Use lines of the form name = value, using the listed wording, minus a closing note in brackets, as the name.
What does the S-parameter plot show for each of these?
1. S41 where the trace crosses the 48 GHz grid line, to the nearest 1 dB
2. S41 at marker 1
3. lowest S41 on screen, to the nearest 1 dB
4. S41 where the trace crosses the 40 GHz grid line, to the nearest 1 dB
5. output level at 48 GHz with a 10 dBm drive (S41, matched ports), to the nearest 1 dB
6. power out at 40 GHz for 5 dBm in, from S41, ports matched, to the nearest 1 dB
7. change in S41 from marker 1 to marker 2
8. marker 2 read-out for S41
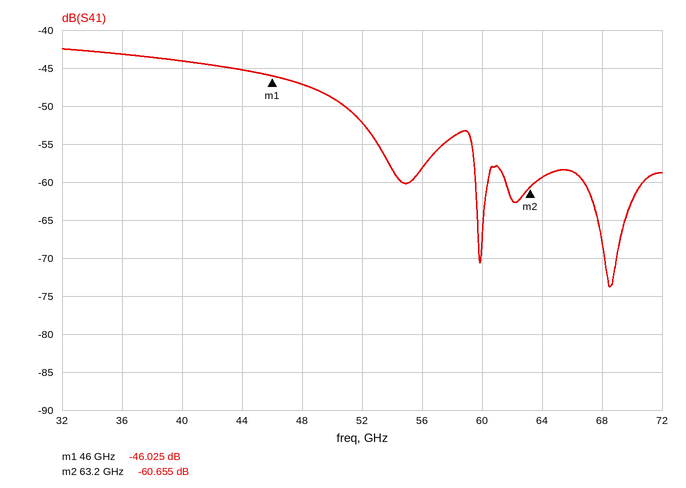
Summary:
S41 where the trace crosses the 48 GHz grid line, to the nearest 1 dB = -47 dB
S41 at marker 1 = -46.025 dB
lowest S41 on screen, to the nearest 1 dB = -74 dB
S41 where the trace crosses the 40 GHz grid line, to the nearest 1 dB = -44 dB
output level at 48 GHz with a 10 dBm drive (S41, matched ports), to the nearest 1 dB = -37 dBm
power out at 40 GHz for 5 dBm in, from S41, ports matched, to the nearest 1 dB = -39 dBm
change in S41 from marker 1 to marker 2 = -14.630 dB
marker 2 read-out for S41 = -60.655 dB
